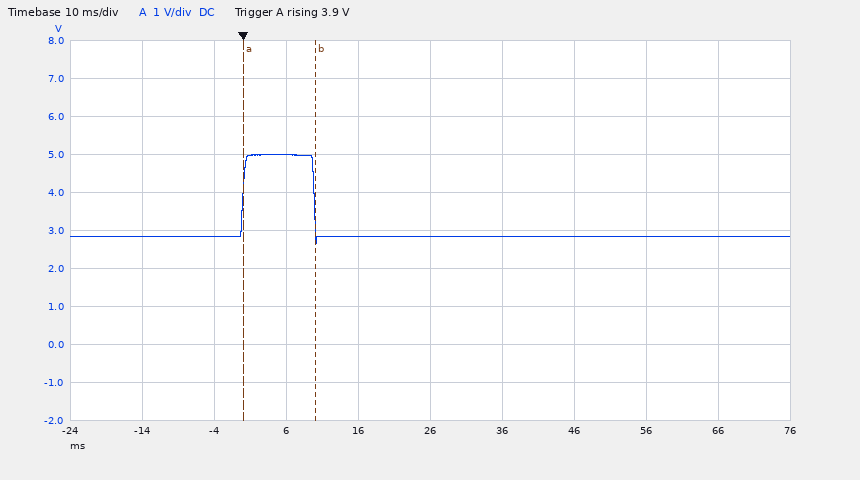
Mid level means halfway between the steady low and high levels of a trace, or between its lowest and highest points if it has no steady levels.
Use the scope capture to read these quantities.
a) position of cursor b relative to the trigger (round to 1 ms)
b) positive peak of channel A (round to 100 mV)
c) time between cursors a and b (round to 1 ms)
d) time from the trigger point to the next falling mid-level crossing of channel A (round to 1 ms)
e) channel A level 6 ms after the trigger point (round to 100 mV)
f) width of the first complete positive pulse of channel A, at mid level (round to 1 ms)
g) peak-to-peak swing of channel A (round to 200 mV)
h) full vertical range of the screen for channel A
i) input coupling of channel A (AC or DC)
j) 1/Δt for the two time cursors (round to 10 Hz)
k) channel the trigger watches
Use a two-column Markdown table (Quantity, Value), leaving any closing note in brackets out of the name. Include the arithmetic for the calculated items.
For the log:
| Quantity | Value |
|---|---|
| position of cursor b relative to the trigger | +10 ms |
| positive peak of channel A | 5.0 V |
| time between cursors a and b | 10 ms |
| time from the trigger point to the next falling mid-level crossing of channel A | 10 ms |
| channel A level 6 ms after the trigger point | 5.0 V |
| width of the first complete positive pulse of channel A, at mid level | 10 ms |
| peak-to-peak swing of channel A | 2.4 V |
| full vertical range of the screen for channel A | 10 V |
| input coupling of channel A | DC |
| 1/Δt for the two time cursors | 1 / 10 ms ≈ 100 Hz |
| channel the trigger watches | channel A |
